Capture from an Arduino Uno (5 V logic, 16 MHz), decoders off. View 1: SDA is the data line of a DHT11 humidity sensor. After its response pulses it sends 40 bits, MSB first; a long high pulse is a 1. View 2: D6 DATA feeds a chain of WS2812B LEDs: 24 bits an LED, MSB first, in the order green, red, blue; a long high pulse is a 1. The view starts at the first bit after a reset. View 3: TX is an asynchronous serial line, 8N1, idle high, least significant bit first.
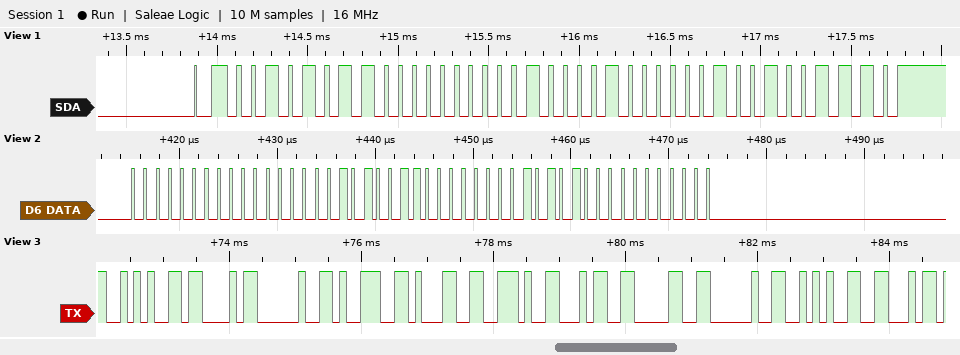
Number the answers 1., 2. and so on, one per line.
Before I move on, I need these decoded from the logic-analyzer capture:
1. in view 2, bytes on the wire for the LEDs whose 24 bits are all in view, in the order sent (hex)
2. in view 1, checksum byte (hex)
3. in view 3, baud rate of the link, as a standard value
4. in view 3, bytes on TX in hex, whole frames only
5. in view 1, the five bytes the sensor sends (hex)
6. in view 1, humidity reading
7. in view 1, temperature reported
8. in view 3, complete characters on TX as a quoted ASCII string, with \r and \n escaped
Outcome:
1. 00 00 53 00 A8 00
2. 0x4E
3. 9600 baud
4. 0x2A 0x43 0x20 0x39 0x31 0x2E 0x34 0x30 0x20 0x2A 0x46
5. 2B 00 21 02 4E
6. 43 %
7. 33.2 °C
8. "*C 91.40 *F"
